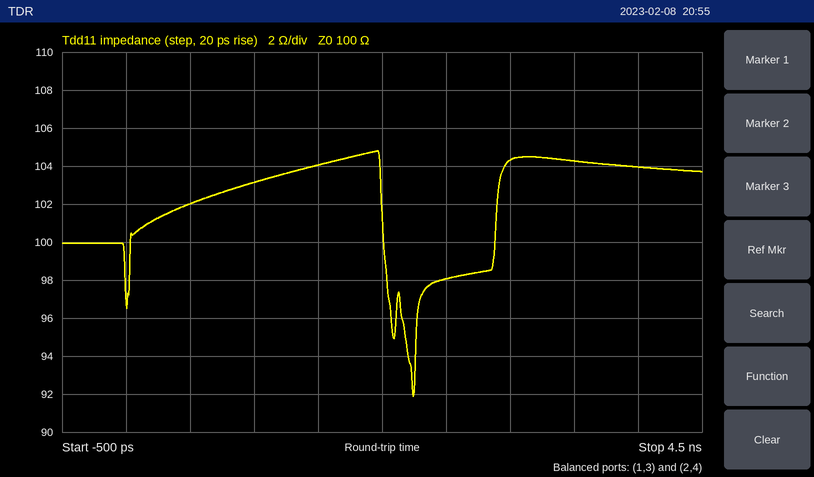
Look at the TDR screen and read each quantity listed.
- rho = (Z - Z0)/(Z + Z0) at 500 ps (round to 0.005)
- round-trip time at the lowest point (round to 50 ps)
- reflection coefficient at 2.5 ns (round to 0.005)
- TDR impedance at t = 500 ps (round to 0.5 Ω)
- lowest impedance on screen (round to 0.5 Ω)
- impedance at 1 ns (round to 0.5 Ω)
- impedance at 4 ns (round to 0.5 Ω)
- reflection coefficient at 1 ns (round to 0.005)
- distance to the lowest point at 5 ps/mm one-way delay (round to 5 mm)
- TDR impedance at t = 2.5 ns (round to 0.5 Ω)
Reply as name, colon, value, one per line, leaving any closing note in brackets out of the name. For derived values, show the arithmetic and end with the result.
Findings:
rho = (Z - Z0)/(Z + Z0) at 500 ps: (102 − 100)/(102 + 100) ≈ +0.010
round-trip time at the lowest point: 2.25 ns
reflection coefficient at 2.5 ns: (98 − 100)/(98 + 100) ≈ -0.010
TDR impedance at t = 500 ps: 102.0 Ω
lowest impedance on screen: 92.0 Ω
impedance at 1 ns: 103.0 Ω
impedance at 4 ns: 104.0 Ω
reflection coefficient at 1 ns: (103 − 100)/(103 + 100) ≈ +0.015
distance to the lowest point at 5 ps/mm one-way delay: 2.25 ns / 2 / 5 ps/mm ≈ 225 mm
TDR impedance at t = 2.5 ns: 98.0 Ω
